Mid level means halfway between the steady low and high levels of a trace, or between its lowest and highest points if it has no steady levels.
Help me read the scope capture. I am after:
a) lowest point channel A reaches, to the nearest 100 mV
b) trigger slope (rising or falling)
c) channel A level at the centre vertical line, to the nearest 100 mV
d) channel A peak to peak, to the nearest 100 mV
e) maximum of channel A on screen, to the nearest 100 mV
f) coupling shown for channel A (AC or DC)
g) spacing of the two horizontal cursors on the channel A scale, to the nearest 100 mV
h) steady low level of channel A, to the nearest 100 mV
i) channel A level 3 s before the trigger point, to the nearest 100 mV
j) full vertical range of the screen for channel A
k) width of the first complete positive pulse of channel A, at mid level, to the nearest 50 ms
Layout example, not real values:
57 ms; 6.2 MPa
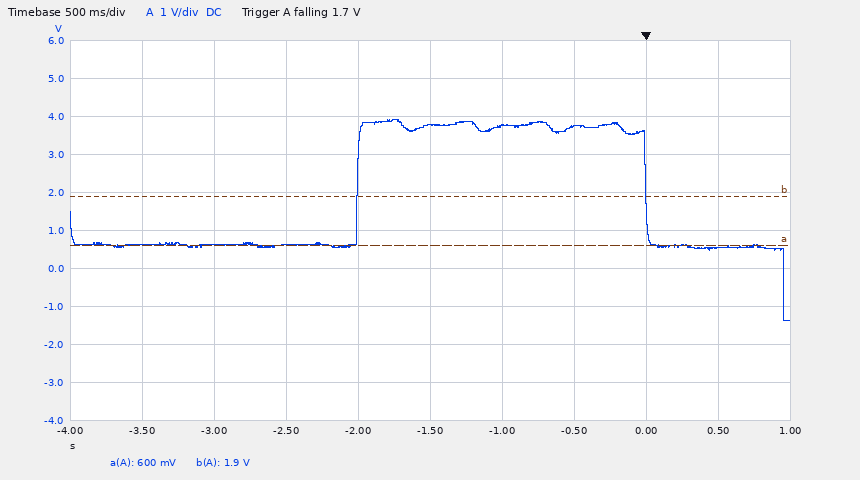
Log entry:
-1.4 V; falling; 3.8 V; 5.3 V; 3.9 V; DC; 1.3 V; 600 mV; 600 mV; 10 V; 2.00 s
